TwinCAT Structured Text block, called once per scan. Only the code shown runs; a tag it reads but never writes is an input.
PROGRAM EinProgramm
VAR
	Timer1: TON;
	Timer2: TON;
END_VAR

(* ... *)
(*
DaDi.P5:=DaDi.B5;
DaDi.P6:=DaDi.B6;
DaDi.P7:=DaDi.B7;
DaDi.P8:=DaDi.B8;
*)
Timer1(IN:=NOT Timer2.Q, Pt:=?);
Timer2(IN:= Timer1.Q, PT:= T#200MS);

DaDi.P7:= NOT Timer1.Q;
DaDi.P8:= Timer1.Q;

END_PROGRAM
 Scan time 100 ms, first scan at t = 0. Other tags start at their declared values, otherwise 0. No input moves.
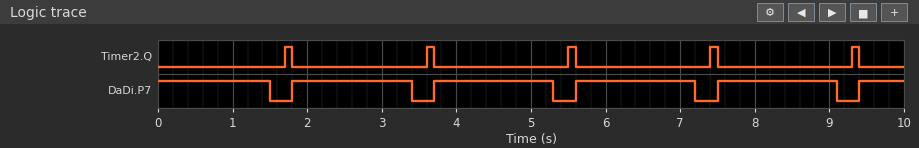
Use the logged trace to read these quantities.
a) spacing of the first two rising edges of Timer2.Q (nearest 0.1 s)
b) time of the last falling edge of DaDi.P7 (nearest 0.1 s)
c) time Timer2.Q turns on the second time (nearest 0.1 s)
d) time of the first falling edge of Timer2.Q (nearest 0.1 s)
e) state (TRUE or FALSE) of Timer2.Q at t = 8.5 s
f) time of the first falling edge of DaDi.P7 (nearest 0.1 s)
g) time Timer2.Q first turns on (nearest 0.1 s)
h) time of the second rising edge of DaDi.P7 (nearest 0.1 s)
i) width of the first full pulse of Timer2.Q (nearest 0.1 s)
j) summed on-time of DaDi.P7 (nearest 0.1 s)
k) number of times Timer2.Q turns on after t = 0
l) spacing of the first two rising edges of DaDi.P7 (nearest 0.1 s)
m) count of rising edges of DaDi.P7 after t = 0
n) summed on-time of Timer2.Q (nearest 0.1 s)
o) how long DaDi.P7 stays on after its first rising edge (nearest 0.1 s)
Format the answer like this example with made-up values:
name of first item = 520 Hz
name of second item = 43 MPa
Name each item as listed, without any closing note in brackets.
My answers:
spacing of the first two rising edges of Timer2.Q = 1.9 s
time of the last falling edge of DaDi.P7 = 9.1 s
time Timer2.Q turns on the second time = 3.6 s
time of the first falling edge of Timer2.Q = 1.8 s
state (TRUE or FALSE) of Timer2.Q at t = 8.5 s = FALSE
time of the first falling edge of DaDi.P7 = 1.5 s
time Timer2.Q first turns on = 1.7 s
time of the second rising edge of DaDi.P7 = 3.7 s
width of the first full pulse of Timer2.Q = 0.1 s
summed on-time of DaDi.P7 = 8.5 s
number of times Timer2.Q turns on after t = 0 = 5
spacing of the first two rising edges of DaDi.P7 = 1.9 s
count of rising edges of DaDi.P7 after t = 0 = 5
summed on-time of Timer2.Q = 0.5 s
how long DaDi.P7 stays on after its first rising edge = 1.6 s
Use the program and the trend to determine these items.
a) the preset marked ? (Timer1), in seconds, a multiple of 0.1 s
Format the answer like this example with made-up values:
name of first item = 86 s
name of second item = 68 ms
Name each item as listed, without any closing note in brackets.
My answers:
the preset marked ? (Timer1), in seconds, a multiple of 0.1 s = 1.5 s
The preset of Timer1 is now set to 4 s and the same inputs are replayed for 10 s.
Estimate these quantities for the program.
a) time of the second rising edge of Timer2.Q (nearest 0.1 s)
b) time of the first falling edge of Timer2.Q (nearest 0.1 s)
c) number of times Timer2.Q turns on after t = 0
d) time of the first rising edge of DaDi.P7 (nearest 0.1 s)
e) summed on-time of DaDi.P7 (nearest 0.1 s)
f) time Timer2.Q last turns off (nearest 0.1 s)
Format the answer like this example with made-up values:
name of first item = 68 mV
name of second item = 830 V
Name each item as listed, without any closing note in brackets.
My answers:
time of the second rising edge of Timer2.Q = 8.6 s
time of the first falling edge of Timer2.Q = 4.3 s
number of times Timer2.Q turns on after t = 0 = 2
time of the first rising edge of DaDi.P7 = 4.3 s
summed on-time of DaDi.P7 = 9.4 s
time Timer2.Q last turns off = 8.7 s
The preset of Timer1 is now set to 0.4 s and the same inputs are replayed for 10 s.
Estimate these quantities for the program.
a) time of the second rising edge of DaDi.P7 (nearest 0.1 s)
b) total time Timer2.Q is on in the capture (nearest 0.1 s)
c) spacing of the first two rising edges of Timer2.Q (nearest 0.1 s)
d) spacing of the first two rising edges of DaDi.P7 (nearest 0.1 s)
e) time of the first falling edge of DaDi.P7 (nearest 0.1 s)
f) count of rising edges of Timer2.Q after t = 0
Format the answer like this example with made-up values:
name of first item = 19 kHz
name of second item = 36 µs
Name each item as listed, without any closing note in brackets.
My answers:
time of the second rising edge of DaDi.P7 = 1.5 s
total time Timer2.Q is on in the capture = 1.2 s
spacing of the first two rising edges of Timer2.Q = 0.8 s
spacing of the first two rising edges of DaDi.P7 = 0.8 s
time of the first falling edge of DaDi.P7 = 0.4 s
count of rising edges of Timer2.Q after t = 0 = 12
